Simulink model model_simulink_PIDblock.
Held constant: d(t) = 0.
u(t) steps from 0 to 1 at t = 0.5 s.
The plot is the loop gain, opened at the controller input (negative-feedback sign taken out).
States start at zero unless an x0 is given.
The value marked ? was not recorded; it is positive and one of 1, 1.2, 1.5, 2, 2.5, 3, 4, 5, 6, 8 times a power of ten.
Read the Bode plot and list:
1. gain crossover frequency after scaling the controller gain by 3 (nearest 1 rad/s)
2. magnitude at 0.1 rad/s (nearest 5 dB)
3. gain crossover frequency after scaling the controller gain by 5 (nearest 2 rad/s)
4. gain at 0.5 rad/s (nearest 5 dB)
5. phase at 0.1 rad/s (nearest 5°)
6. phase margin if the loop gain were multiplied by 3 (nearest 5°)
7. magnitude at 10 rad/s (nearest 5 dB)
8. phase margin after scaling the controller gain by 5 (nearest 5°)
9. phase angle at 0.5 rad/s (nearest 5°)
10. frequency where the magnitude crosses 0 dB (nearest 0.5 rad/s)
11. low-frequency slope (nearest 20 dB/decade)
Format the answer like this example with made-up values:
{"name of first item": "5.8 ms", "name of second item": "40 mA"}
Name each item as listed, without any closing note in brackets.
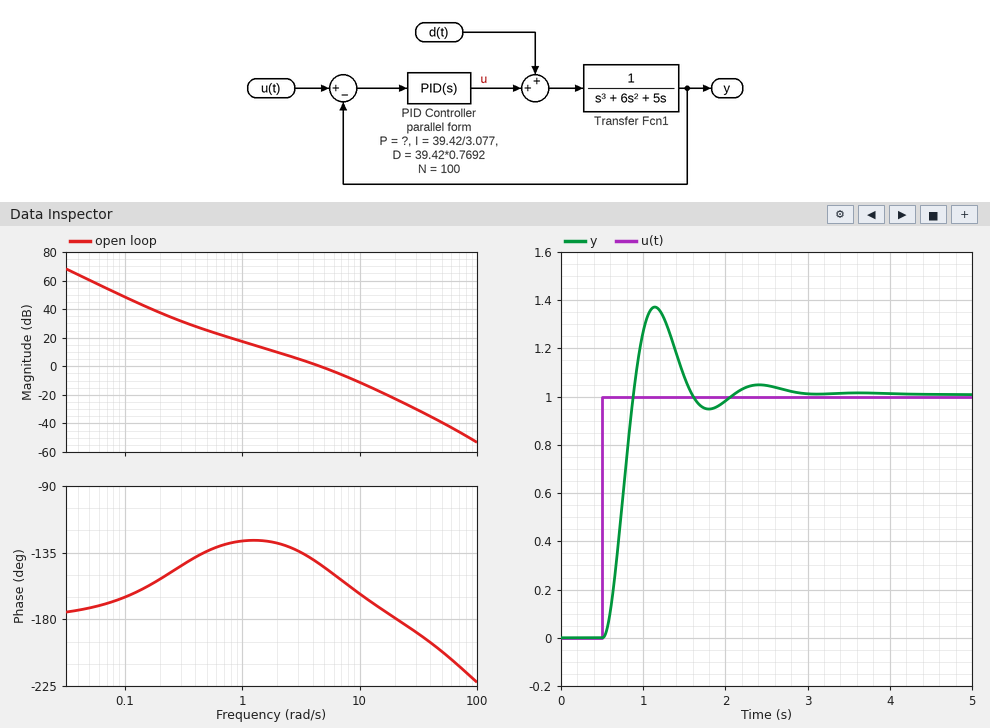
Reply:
{"gain crossover frequency after scaling the controller gain by 3": "9 rad/s", "magnitude at 0.1 rad/s": "50 dB", "gain crossover frequency after scaling the controller gain by 5": "12 rad/s", "gain at 0.5 rad/s": "25 dB", "phase at 0.1 rad/s": "-165°", "phase margin if the loop gain were multiplied by 3": "20°", "magnitude at 10 rad/s": "-10 dB", "phase margin after scaling the controller gain by 5": "15°", "phase angle at 0.5 rad/s": "-135°", "frequency where the magnitude crosses 0 dB": "4.5 rad/s", "low-frequency slope": "-40 dB/decade"}
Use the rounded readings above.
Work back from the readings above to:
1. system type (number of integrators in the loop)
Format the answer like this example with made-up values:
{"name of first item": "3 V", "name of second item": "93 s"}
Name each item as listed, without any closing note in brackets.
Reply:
{"system type": "2"}
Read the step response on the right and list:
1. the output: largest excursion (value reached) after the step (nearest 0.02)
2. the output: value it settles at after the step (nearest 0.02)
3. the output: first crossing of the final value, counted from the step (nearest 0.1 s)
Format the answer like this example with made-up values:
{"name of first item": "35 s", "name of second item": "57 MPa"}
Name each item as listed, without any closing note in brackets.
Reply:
{"the output: largest excursion (value reached) after the step": "1.38", "the output: value it settles at after the step": "1.00", "the output: first crossing of the final value, counted from the step": "0.4 s"}
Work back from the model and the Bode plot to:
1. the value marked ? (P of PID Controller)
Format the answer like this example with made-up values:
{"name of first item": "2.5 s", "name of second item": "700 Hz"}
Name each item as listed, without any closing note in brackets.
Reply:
{"the value marked ?": "50"}
